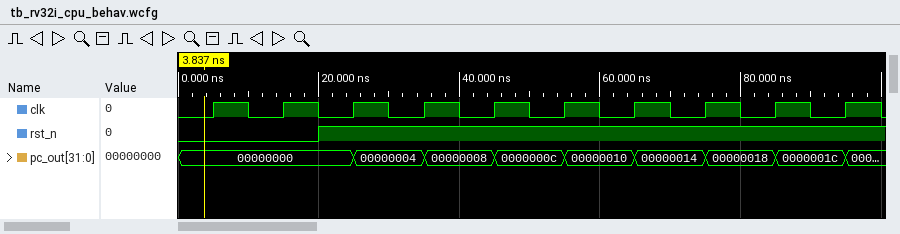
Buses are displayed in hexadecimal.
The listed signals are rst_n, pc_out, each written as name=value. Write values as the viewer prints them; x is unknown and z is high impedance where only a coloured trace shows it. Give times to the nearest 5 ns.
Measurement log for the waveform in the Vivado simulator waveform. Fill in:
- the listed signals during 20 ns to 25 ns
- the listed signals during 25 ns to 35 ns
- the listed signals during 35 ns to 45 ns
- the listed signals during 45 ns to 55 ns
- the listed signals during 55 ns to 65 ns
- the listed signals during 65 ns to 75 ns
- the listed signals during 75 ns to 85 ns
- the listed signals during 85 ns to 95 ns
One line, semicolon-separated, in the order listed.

rst_n=1, pc_out=00000000; rst_n=1, pc_out=00000004; rst_n=1, pc_out=00000008; rst_n=1, pc_out=0000000c; rst_n=1, pc_out=00000010; rst_n=1, pc_out=00000014; rst_n=1, pc_out=00000018; rst_n=1, pc_out=0000001c
